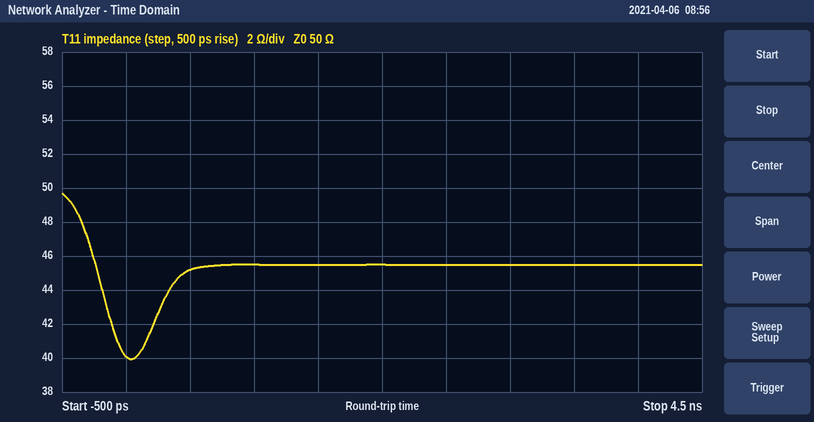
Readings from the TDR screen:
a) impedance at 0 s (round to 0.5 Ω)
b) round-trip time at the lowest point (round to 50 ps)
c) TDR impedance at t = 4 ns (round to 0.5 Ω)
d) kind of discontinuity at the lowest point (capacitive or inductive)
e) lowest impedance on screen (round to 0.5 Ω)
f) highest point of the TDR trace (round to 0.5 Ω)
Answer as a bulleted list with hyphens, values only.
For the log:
- 40.0 Ω
- 50 ps
- 45.5 Ω
- capacitive
- 40.0 Ω
- 49.5 Ω
